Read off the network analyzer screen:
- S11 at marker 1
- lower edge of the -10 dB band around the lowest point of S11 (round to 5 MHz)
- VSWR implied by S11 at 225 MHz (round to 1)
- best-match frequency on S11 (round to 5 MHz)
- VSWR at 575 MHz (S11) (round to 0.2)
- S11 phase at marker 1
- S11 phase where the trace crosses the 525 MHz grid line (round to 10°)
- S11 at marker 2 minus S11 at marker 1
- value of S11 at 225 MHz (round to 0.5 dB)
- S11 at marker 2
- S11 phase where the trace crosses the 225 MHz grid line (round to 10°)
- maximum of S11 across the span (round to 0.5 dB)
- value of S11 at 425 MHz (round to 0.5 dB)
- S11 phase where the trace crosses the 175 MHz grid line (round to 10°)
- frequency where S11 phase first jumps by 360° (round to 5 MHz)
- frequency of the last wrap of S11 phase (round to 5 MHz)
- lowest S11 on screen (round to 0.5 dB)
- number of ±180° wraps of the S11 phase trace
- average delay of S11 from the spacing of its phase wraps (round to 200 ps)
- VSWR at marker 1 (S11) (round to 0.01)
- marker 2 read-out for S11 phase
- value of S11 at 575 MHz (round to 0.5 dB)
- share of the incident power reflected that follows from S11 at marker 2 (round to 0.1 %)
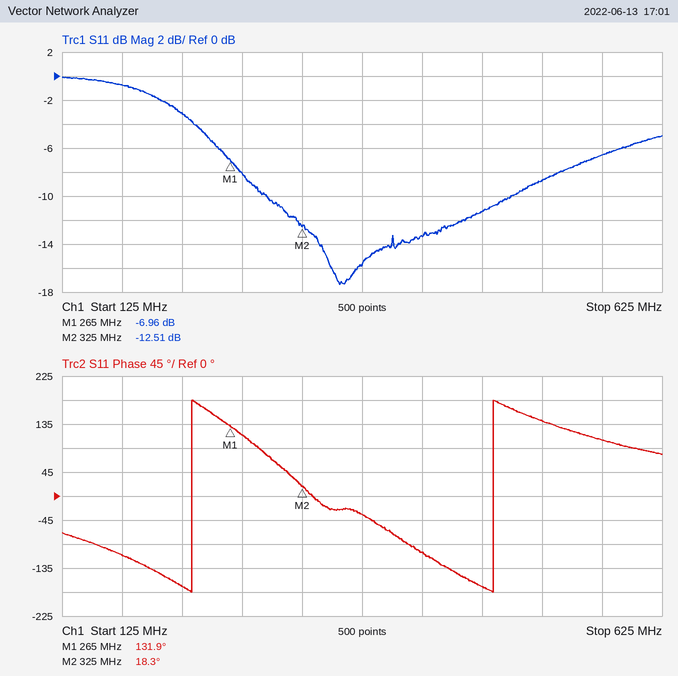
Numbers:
-6.96 dB
295 MHz
6
355 MHz
2.8
131.9°
140°
-5.55 dB
-3.0 dB
-12.51 dB
-170°
0.0 dB
-13.5 dB
-110°
235 MHz
485 MHz
-17.5 dB
2
4.0 ns
2.63
18.3°
-6.5 dB
5.6 %
